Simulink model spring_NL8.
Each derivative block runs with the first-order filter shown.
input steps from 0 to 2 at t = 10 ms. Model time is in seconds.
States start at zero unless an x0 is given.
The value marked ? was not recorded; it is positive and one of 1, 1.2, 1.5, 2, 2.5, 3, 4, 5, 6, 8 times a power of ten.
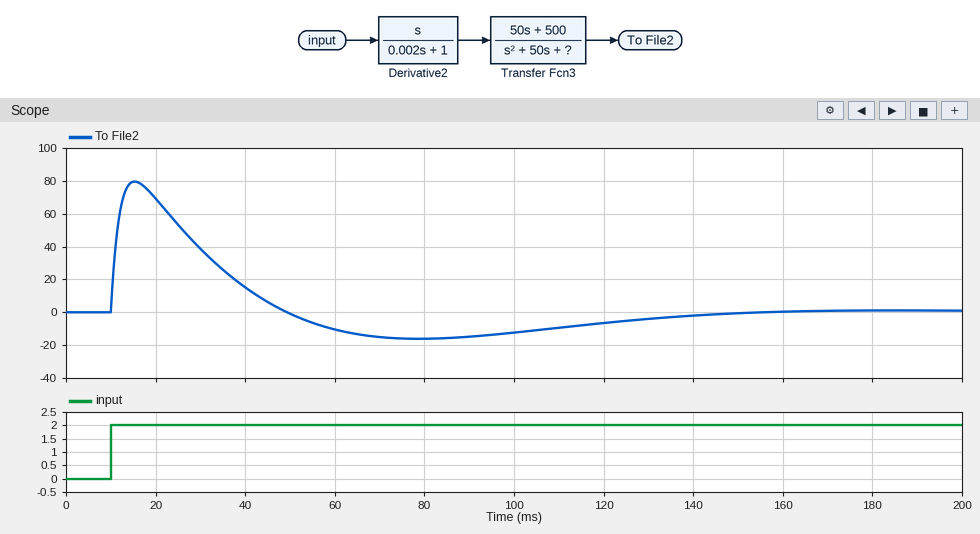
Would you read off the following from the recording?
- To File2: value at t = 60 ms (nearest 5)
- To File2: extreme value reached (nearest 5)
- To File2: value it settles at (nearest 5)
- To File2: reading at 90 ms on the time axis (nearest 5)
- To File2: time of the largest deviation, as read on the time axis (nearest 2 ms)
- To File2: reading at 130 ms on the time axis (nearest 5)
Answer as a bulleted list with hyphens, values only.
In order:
- -10
- 80
- 0
- -15
- 16 ms
- -5
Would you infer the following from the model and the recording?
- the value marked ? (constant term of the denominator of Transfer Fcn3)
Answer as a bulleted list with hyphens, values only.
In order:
- 1500
